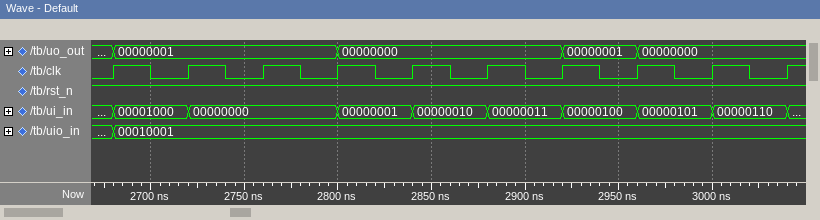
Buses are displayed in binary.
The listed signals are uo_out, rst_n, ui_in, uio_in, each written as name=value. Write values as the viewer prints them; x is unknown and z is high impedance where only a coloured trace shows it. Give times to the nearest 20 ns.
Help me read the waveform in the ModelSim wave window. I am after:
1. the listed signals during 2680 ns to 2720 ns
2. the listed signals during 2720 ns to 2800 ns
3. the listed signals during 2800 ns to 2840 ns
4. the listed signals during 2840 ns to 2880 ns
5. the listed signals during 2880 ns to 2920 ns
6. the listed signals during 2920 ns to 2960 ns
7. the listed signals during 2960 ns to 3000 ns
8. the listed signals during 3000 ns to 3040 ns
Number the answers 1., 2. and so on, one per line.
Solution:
1. uo_out=00000001, rst_n=1, ui_in=00001000, uio_in=00010001
2. uo_out=00000001, rst_n=1, ui_in=00000000, uio_in=00010001
3. uo_out=00000000, rst_n=1, ui_in=00000001, uio_in=00010001
4. uo_out=00000000, rst_n=1, ui_in=00000010, uio_in=00010001
5. uo_out=00000000, rst_n=1, ui_in=00000011, uio_in=00010001
6. uo_out=00000001, rst_n=1, ui_in=00000100, uio_in=00010001
7. uo_out=00000000, rst_n=1, ui_in=00000101, uio_in=00010001
8. uo_out=00000000, rst_n=1, ui_in=00000110, uio_in=00010001
